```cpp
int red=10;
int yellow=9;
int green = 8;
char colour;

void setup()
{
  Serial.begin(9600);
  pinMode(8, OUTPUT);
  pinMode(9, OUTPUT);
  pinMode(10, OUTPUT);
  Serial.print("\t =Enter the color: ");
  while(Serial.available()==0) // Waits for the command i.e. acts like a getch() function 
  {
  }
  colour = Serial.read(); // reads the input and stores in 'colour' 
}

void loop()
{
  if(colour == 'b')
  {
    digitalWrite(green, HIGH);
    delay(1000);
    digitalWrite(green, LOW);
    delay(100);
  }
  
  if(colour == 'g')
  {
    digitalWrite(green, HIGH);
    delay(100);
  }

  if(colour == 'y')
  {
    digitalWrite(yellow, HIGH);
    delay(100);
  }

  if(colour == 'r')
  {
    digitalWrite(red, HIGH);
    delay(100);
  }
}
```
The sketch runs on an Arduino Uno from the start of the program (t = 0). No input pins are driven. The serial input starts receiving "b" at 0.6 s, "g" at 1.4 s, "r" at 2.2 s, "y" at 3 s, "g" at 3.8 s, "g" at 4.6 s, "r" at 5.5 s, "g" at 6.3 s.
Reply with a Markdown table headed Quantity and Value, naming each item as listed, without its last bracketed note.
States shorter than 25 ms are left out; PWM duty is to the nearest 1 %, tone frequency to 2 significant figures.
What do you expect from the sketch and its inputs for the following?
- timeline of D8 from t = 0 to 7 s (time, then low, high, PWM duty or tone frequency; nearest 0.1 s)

| Quantity | Value |
|---|---|
| timeline of D8 from t = 0 to 7 s | 0 s low; 0.6 s high; 1.6 s low; 1.7 s high; 2.7 s low; 2.8 s high; 3.8 s low; 3.9 s high; 4.9 s low; 5 s high; 6 s low; 6.1 s high |
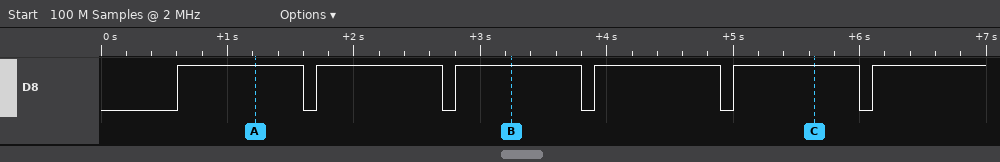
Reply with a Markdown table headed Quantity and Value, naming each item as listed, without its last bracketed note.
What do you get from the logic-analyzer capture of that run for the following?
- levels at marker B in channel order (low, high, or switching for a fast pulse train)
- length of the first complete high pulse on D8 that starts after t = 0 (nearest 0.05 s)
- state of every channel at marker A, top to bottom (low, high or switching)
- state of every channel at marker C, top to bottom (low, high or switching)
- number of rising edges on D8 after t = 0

| Quantity | Value |
|---|---|
| levels at marker B in channel order | D8 high |
| length of the first complete high pulse on D8 that starts after t = 0 | 1.00 s |
| state of every channel at marker A, top to bottom | D8 high |
| state of every channel at marker C, top to bottom | D8 high |
| number of rising edges on D8 after t = 0 | 6 |
